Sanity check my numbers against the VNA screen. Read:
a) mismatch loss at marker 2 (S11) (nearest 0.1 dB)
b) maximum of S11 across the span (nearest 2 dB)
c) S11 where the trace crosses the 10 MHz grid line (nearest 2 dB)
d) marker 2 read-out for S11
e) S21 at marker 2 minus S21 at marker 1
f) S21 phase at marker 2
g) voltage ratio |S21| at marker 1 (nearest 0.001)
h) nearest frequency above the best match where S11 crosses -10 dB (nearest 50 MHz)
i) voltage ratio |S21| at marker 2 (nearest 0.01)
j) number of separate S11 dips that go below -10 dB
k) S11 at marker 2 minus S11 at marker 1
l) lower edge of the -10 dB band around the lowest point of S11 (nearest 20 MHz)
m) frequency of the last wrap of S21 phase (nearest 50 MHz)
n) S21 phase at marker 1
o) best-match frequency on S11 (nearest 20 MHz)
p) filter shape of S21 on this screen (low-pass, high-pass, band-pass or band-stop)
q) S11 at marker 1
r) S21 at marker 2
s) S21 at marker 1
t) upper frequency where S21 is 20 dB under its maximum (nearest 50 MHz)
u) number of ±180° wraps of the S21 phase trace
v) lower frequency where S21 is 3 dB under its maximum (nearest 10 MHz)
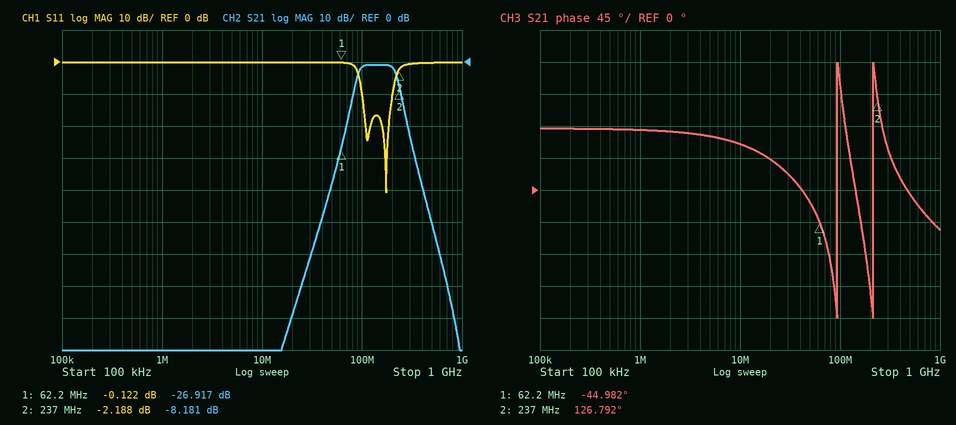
4.0 dB
0 dB
0 dB
-2.188 dB
18.736 dB
126.792°
0.045
200 MHz
0.39
2
-2.066 dB
100 MHz
200 MHz
-44.982°
180 MHz
band-pass
-0.122 dB
-8.181 dB
-26.917 dB
300 MHz
2
90 MHz
